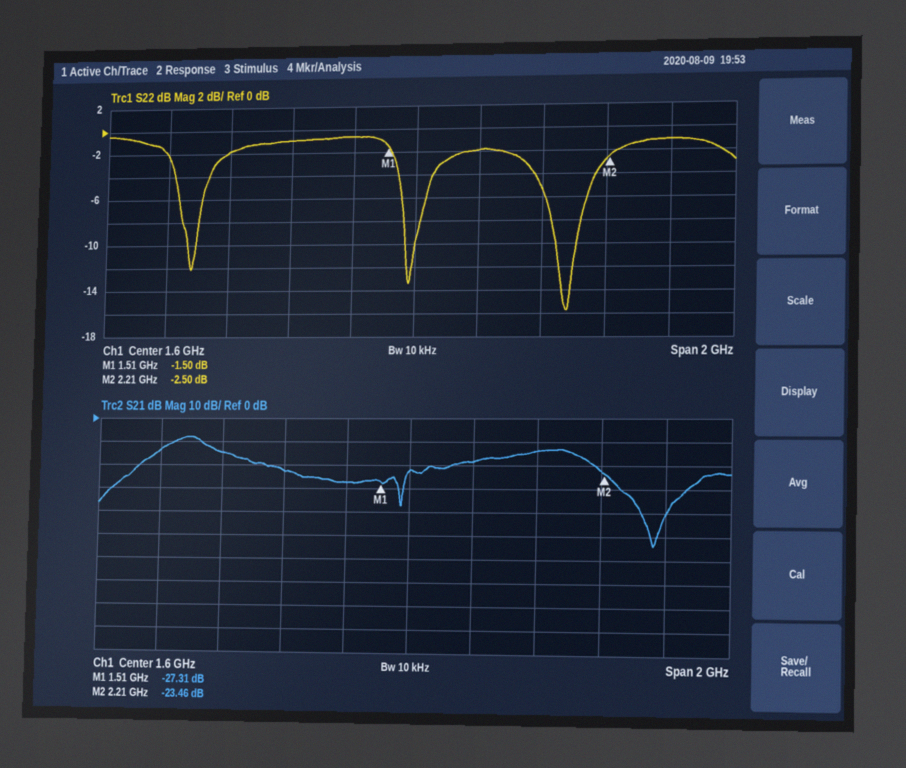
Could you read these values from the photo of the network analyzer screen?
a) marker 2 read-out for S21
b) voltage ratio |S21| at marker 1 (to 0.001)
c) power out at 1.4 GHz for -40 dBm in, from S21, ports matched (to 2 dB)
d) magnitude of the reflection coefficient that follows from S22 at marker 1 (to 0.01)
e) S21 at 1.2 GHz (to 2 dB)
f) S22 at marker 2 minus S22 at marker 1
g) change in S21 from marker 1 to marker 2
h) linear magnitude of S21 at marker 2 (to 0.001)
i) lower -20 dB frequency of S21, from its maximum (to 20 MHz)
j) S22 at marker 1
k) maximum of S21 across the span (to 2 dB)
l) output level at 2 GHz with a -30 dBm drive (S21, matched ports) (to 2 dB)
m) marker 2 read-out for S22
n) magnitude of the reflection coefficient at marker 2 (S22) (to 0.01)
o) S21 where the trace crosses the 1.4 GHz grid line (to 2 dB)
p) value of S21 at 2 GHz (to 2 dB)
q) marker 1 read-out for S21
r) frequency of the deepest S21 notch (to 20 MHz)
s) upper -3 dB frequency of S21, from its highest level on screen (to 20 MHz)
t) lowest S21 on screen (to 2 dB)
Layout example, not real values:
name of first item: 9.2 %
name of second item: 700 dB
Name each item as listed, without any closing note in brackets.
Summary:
marker 2 read-out for S21: -23.46 dB
voltage ratio |S21| at marker 1: 0.043
power out at 1.4 GHz for -40 dBm in, from S21, ports matched: -68 dBm
magnitude of the reflection coefficient that follows from S22 at marker 1: 0.84
S21 at 1.2 GHz: -22 dB
S22 at marker 2 minus S22 at marker 1: -1.00 dB
change in S21 from marker 1 to marker 2: 3.85 dB
linear magnitude of S21 at marker 2: 0.067
lower -20 dB frequency of S21, from its maximum: 660 MHz
S22 at marker 1: -1.50 dB
maximum of S21 across the span: -8 dB
output level at 2 GHz with a -30 dBm drive (S21, matched ports): -44 dBm
marker 2 read-out for S22: -2.50 dB
magnitude of the reflection coefficient at marker 2 (S22): 0.75
S21 where the trace crosses the 1.4 GHz grid line: -28 dB
value of S21 at 2 GHz: -14 dB
marker 1 read-out for S21: -27.31 dB
frequency of the deepest S21 notch: 2.36 GHz
upper -3 dB frequency of S21, from its highest level on screen: 940 MHz
lowest S21 on screen: -54 dB
